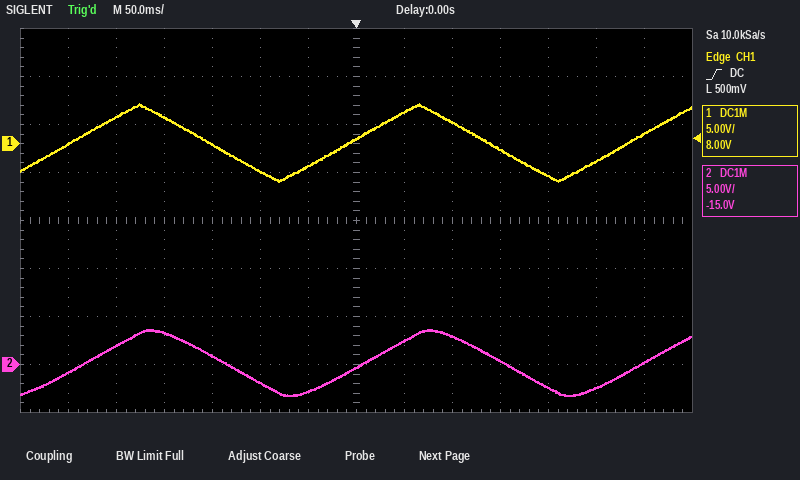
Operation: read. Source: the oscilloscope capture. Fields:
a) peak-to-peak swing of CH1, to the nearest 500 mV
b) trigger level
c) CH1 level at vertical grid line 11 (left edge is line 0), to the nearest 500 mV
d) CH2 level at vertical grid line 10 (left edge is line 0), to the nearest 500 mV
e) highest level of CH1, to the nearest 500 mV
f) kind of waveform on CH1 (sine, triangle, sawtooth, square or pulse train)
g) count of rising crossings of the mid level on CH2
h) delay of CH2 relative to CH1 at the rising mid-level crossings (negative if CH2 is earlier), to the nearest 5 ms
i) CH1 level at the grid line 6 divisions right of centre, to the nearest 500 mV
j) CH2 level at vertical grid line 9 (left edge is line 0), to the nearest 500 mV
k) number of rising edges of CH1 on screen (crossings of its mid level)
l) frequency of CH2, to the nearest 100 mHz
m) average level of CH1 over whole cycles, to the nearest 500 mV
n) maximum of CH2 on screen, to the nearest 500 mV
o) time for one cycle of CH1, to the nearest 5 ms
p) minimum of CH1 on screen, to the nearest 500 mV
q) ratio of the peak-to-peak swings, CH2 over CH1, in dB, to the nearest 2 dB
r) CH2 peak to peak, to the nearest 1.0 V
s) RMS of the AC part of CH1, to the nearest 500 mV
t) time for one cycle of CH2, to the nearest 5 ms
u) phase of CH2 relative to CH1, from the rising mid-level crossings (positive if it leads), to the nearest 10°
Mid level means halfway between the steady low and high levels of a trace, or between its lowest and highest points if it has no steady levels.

8.0 V
500 mV
-3.5 V
500 mV
4.0 V
triangle
3
+15 ms
1.0 V
3.0 V
3
3.4 Hz
0.0 V
3.5 V
290 ms
-4.0 V
-2 dB
7.0 V
2.5 V
290 ms
-20°
